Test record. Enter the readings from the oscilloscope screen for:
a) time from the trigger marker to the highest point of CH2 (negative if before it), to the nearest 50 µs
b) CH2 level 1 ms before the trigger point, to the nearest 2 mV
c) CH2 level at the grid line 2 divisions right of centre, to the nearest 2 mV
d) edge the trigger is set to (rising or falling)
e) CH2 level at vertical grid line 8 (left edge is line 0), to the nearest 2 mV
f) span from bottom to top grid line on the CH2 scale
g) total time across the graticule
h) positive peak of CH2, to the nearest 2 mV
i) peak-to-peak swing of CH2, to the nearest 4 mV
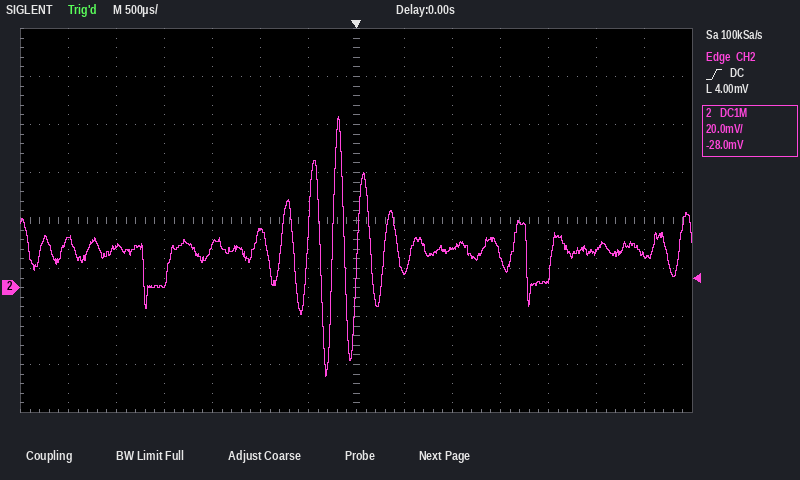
-200 µs
24 mV
16 mV
rising
6 mV
160 mV
7 ms
72 mV
108 mV
